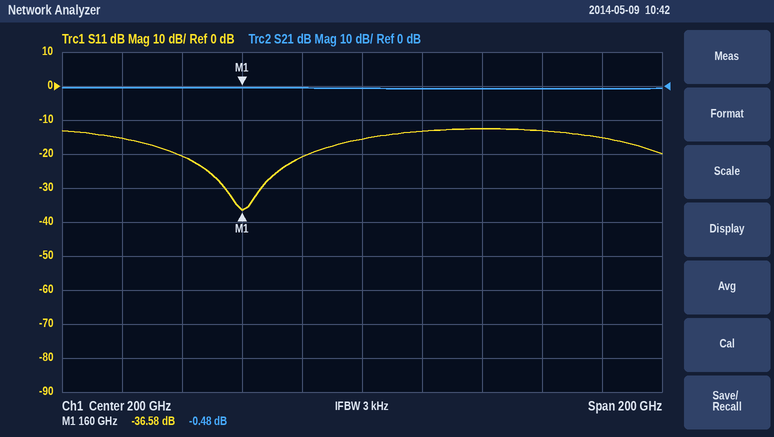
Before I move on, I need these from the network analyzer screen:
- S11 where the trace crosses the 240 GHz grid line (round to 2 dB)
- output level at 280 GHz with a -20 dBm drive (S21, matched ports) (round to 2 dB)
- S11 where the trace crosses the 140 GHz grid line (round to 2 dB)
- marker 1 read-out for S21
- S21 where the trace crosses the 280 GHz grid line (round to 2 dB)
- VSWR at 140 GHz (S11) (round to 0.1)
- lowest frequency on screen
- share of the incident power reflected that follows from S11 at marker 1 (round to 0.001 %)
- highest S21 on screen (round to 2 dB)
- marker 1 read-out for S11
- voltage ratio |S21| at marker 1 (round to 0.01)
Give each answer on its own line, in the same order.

-12 dB
-20 dBm
-20 dB
-0.48 dB
0 dB
1.2
100 GHz
0.022 %
0 dB
-36.58 dB
0.95
